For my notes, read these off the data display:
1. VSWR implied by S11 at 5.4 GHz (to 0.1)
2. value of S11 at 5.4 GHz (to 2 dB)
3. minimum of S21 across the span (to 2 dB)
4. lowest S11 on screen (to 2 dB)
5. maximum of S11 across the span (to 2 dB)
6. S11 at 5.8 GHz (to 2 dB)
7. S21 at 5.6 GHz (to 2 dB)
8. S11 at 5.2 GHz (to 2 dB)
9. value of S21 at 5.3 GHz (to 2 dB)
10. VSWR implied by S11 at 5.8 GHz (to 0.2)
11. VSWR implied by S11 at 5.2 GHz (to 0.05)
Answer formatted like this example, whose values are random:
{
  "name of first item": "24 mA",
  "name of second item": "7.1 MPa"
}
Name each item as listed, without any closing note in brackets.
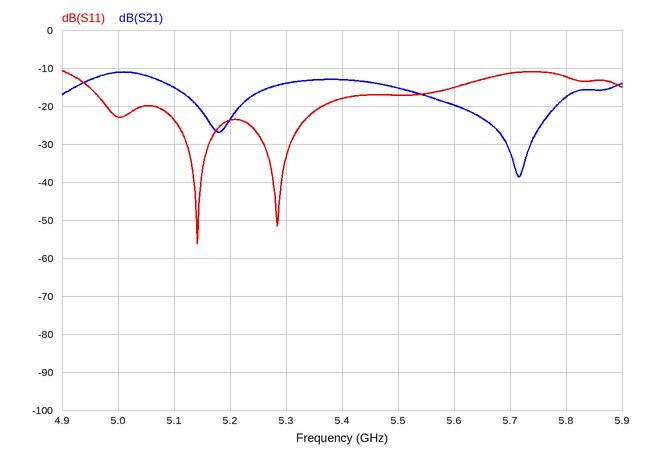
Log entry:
{
  "VSWR implied by S11 at 5.4 GHz": "1.3",
  "value of S11 at 5.4 GHz": "-18 dB",
  "minimum of S21 across the span": "-38 dB",
  "lowest S11 on screen": "-56 dB",
  "maximum of S11 across the span": "-10 dB",
  "S11 at 5.8 GHz": "-12 dB",
  "S21 at 5.6 GHz": "-20 dB",
  "S11 at 5.2 GHz": "-24 dB",
  "value of S21 at 5.3 GHz": "-14 dB",
  "VSWR implied by S11 at 5.8 GHz": "1.6",
  "VSWR implied by S11 at 5.2 GHz": "1.15"
}
